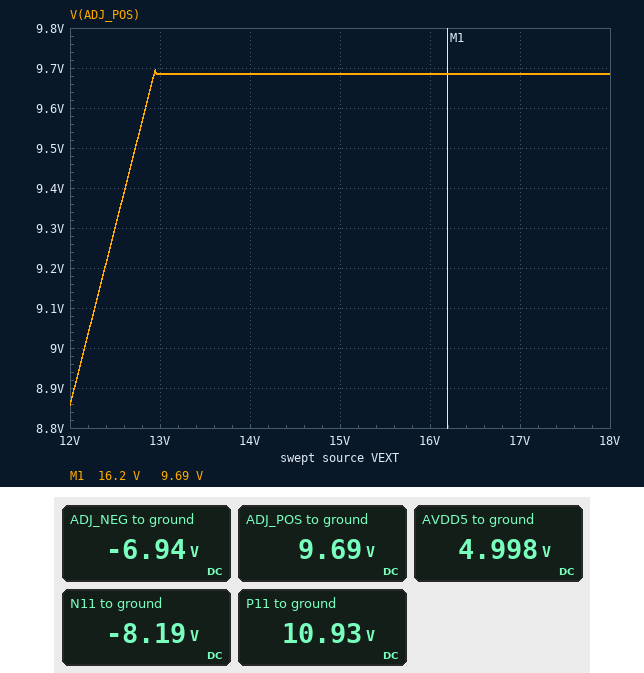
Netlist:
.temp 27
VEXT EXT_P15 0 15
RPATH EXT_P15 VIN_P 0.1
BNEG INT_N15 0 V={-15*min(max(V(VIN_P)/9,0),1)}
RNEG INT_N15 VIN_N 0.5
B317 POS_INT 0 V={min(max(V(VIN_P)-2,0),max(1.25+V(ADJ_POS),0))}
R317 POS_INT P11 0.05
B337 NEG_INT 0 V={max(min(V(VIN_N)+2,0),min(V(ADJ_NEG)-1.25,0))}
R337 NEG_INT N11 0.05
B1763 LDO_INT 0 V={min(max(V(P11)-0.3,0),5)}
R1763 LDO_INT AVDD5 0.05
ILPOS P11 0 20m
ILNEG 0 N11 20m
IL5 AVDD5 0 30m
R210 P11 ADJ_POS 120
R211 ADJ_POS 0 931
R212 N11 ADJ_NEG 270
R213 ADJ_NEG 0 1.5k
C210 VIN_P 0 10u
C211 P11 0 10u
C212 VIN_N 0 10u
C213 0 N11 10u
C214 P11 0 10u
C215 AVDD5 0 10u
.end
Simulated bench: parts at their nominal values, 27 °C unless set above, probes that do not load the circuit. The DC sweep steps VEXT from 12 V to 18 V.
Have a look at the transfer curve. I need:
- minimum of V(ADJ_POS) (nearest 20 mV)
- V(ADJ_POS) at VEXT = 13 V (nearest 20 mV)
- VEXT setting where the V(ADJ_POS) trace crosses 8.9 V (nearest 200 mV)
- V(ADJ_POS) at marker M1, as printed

8.86 V
9.68 V
12.0 V
9.69 V
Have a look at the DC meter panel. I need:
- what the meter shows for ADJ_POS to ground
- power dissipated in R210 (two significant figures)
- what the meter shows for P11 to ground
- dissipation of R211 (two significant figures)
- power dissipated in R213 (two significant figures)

9.69 V
13 mW
10.93 V
100 mW
32 mW
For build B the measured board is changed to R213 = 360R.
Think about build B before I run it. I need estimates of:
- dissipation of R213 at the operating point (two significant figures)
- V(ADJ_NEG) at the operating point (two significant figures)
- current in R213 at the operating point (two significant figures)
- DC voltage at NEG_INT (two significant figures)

7.7 mW
-1.7 V
4.6 mA
-2.9 V
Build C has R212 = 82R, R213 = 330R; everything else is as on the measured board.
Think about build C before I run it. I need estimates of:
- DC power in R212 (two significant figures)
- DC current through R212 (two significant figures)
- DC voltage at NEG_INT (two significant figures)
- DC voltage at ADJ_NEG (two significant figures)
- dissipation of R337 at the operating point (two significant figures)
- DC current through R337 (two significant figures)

19 mW
15 mA
-6.3 V
-5.0 V
62 µW
35 mA
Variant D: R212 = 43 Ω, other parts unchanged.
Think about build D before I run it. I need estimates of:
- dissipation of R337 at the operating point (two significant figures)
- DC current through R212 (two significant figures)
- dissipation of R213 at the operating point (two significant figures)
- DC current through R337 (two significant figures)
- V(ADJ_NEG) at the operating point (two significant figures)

40 µW
8.4 mA
110 mW
28 mA
-13 V
